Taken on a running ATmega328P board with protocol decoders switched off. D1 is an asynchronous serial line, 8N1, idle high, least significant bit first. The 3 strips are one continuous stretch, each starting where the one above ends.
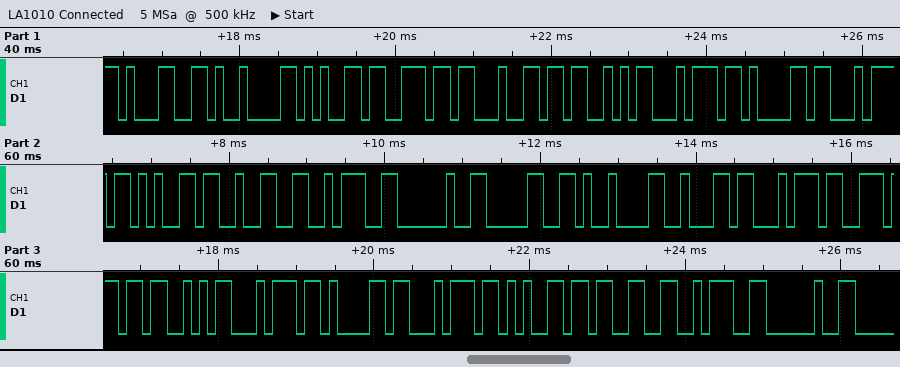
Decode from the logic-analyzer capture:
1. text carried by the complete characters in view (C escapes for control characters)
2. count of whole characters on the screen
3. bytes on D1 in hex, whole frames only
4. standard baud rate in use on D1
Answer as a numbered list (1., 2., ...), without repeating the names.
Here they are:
1. "1\tendState2: 0\tbtnState3: "
2. 26
3. 31 09 65 6E 64 53 74 61 74 65 32 3A 20 30 09 62 74 6E 53 74 61 74 65 33 3A 20
4. 9600 baud
